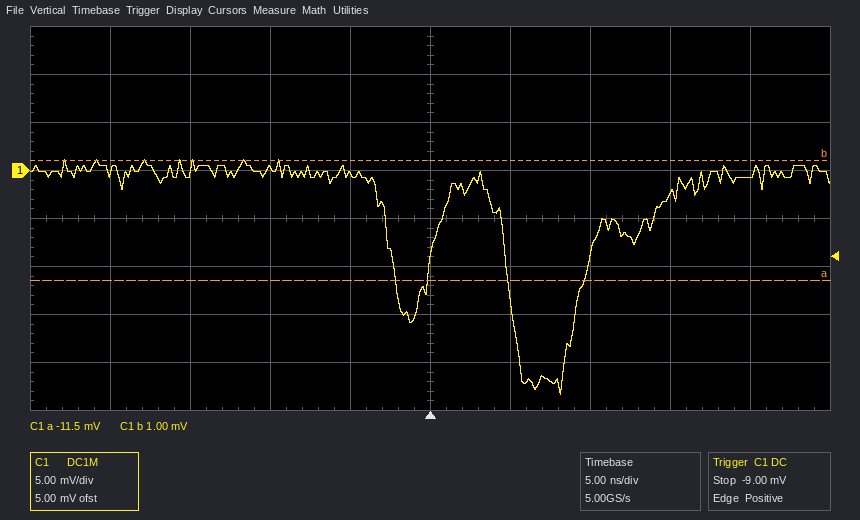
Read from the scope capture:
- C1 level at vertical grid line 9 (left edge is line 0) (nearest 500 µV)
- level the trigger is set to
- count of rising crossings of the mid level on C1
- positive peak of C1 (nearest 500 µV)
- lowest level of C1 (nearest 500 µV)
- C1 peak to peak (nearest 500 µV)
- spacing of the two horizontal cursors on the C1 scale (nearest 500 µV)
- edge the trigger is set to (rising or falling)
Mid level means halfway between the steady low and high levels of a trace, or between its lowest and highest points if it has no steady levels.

-500 µV
-9.00 mV
2
1.0 mV
-23.5 mV
24.5 mV
12.5 mV
rising
